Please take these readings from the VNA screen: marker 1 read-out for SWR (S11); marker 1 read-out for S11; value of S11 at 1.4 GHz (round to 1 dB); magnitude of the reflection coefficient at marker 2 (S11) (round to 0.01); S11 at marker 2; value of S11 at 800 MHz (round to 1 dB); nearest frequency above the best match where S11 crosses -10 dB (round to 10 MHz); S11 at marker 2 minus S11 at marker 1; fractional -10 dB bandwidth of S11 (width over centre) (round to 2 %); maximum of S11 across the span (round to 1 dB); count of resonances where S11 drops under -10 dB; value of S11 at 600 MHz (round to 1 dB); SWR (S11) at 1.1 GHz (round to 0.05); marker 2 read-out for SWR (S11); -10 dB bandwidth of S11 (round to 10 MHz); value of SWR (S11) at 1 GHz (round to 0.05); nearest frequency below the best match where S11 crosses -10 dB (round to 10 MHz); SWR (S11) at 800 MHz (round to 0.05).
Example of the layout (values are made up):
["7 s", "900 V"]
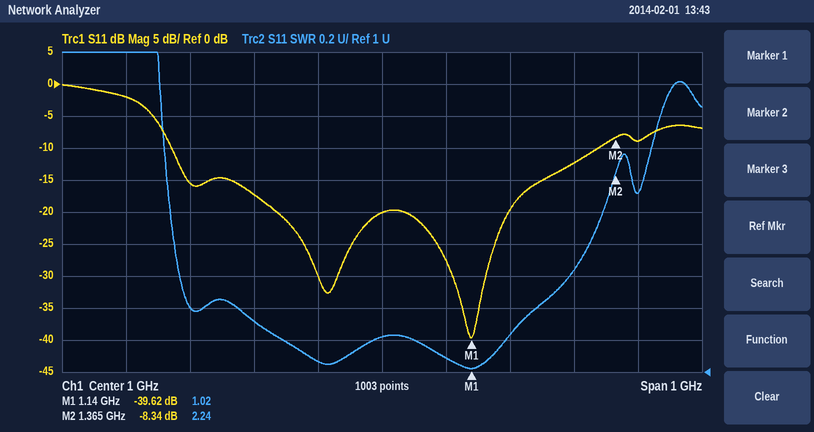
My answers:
["1.02", "-39.62 dB", "-9 dB", "0.38", "-8.34 dB", "-17 dB", "1.34 GHz", "31.28 dB", "66 %", "0 dB", "2", "-2 dB", "1.10", "2.24", "670 MHz", "1.20", "670 MHz", "1.30"]
